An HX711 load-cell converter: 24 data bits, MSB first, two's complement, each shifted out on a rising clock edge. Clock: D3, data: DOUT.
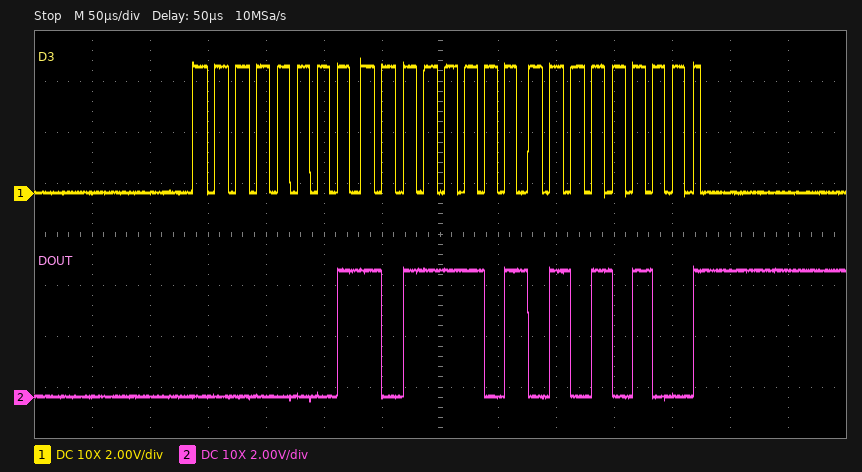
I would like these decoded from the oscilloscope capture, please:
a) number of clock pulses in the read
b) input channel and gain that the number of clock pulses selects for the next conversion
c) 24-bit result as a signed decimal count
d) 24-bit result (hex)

25
channel A, gain 128
114004
0x01BD54
